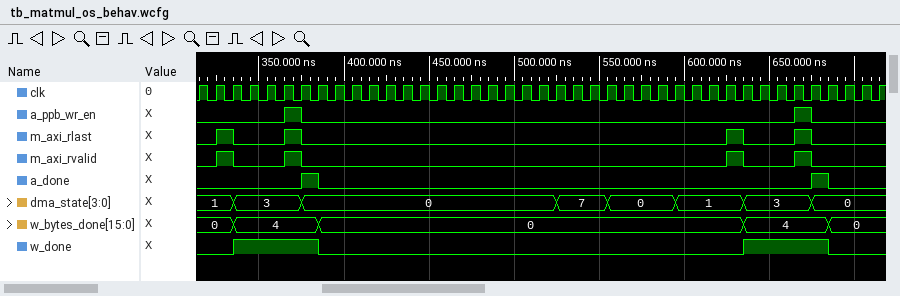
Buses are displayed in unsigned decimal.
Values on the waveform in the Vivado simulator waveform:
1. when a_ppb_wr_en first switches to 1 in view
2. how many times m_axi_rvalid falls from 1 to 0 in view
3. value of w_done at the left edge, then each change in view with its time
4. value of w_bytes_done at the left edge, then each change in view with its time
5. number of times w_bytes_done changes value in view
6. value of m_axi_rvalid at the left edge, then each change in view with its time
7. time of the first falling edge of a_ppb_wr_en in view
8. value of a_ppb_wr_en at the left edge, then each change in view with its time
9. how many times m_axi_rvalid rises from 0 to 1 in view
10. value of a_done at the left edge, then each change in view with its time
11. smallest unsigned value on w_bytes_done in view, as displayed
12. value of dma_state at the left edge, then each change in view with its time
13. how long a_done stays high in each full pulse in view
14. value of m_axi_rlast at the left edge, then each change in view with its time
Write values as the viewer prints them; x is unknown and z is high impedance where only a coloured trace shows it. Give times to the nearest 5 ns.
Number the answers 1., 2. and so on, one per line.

1. 365 ns
2. 4
3. 0, 1 at 335 ns, 0 at 385 ns, 1 at 635 ns, 0 at 685 ns
4. 0, 4 at 335 ns, 0 at 385 ns, 4 at 635 ns, 0 at 685 ns
5. 4
6. 0, 1 at 325 ns, 0 at 335 ns, 1 at 365 ns, 0 at 375 ns, 1 at 625 ns, 0 at 635 ns, 1 at 665 ns, 0 at 675 ns
7. 375 ns
8. 0, 1 at 365 ns, 0 at 375 ns, 1 at 665 ns, 0 at 675 ns
9. 4
10. 0, 1 at 375 ns, 0 at 385 ns, 1 at 675 ns, 0 at 685 ns
11. 0
12. 1, 3 at 335 ns, 0 at 375 ns, 7 at 525 ns, 0 at 555 ns, 1 at 595 ns, 3 at 635 ns, 0 at 675 ns
13. 10 ns, 10 ns
14. 0, 1 at 325 ns, 0 at 335 ns, 1 at 365 ns, 0 at 375 ns, 1 at 625 ns, 0 at 635 ns, 1 at 665 ns, 0 at 675 ns
